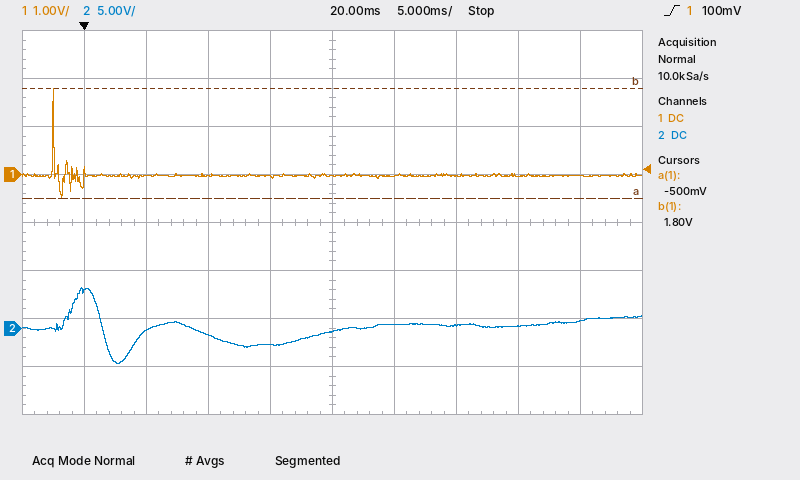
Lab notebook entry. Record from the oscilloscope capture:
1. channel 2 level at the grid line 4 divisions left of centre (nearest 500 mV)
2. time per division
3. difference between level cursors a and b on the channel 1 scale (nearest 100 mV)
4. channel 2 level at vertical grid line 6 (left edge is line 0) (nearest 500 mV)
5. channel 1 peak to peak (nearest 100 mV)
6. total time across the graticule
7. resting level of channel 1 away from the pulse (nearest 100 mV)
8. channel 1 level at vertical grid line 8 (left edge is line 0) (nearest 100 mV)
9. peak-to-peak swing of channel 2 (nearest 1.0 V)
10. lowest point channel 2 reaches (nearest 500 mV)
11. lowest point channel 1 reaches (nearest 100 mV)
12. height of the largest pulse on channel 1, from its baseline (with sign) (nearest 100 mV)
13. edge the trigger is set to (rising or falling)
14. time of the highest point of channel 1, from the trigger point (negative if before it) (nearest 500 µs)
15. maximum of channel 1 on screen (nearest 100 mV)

4.0 V
5 ms
2.3 V
500 mV
2.3 V
50 ms
0.0 V
0.0 V
8.0 V
-3.5 V
-500 mV
+1.8 V
rising
-2.5 ms
1.8 V
